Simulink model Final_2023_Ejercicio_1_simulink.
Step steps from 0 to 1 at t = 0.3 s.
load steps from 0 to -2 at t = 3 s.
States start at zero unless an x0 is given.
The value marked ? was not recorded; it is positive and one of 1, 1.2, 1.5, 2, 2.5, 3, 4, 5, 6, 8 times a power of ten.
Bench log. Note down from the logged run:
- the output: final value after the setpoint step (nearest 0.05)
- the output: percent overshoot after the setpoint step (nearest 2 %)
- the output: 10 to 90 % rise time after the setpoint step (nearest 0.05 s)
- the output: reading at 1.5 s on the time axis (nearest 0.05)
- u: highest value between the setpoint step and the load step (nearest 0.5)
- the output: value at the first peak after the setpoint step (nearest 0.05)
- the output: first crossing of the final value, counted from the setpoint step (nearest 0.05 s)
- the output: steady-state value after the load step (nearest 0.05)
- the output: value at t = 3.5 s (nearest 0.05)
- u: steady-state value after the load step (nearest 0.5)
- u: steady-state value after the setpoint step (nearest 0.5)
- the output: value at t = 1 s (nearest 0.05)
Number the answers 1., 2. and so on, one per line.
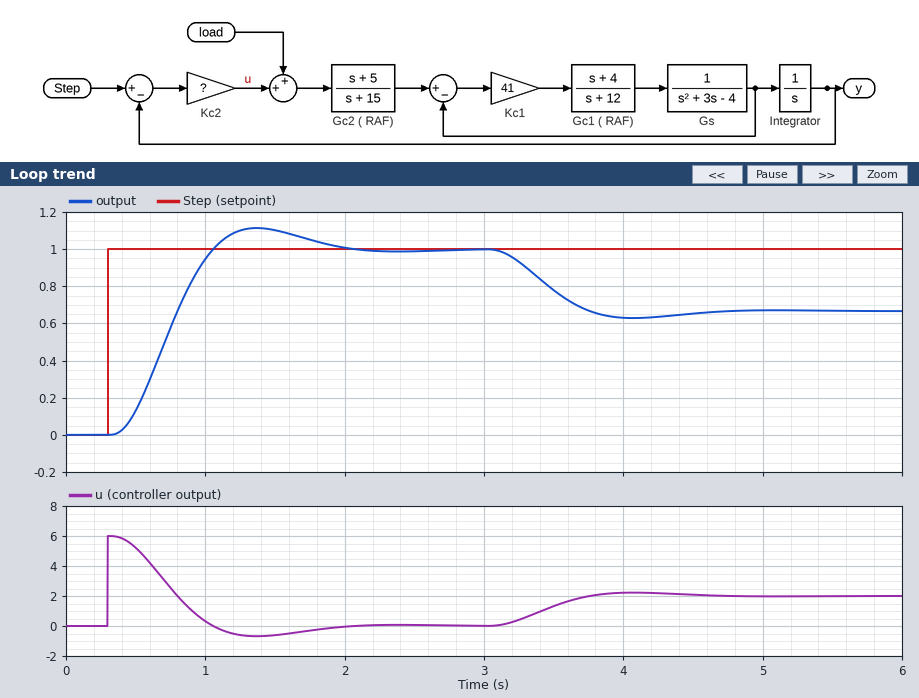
1. 1.00
2. 12 %
3. 0.50 s
4. 1.10
5. 6.0
6. 1.10
7. 0.75 s
8. 0.65
9. 0.80
10. 2.0
11. 0.0
12. 0.95
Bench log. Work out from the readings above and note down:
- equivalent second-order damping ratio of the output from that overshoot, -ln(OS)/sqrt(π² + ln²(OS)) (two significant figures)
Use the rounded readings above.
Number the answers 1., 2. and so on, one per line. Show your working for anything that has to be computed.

1. ln(0.12) = -2.120; 2.120 / sqrt(9.870 + 4.496) = 0.56
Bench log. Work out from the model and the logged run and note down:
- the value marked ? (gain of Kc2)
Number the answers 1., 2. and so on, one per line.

1. 6
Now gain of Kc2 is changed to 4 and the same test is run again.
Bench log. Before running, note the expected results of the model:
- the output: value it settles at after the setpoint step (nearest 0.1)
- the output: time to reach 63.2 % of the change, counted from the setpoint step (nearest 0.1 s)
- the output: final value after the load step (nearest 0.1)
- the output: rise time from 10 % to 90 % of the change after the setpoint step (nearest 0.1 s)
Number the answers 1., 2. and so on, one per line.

1. 1.0
2. 0.6 s
3. 0.5
4. 0.7 s
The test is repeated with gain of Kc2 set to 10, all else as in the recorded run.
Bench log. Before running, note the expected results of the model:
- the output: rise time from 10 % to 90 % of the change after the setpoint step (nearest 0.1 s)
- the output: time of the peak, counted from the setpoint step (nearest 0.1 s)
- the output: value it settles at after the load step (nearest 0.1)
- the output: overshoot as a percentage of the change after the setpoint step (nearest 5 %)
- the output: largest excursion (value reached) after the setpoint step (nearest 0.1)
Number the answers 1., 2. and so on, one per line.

1. 0.3 s
2. 0.8 s
3. 0.8
4. 25 %
5. 1.3
